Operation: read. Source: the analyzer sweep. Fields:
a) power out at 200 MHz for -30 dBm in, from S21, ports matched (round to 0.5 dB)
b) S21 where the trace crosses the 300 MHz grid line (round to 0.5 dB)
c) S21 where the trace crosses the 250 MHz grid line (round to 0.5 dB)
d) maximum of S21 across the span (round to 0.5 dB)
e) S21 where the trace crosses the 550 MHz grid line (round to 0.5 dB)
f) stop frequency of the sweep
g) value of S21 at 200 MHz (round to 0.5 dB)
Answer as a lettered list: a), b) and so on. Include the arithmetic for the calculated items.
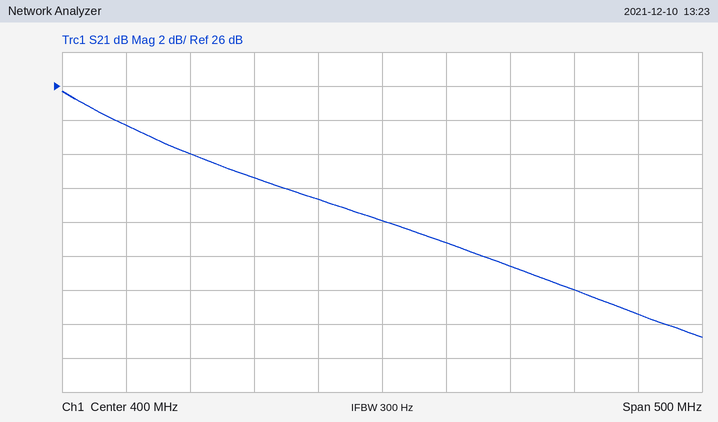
a) -30 dBm + (23.5 dB) = -6.5 dBm
b) 20.5 dB
c) 22.0 dB
d) 25.5 dB
e) 14.0 dB
f) 650 MHz
g) 23.5 dB
